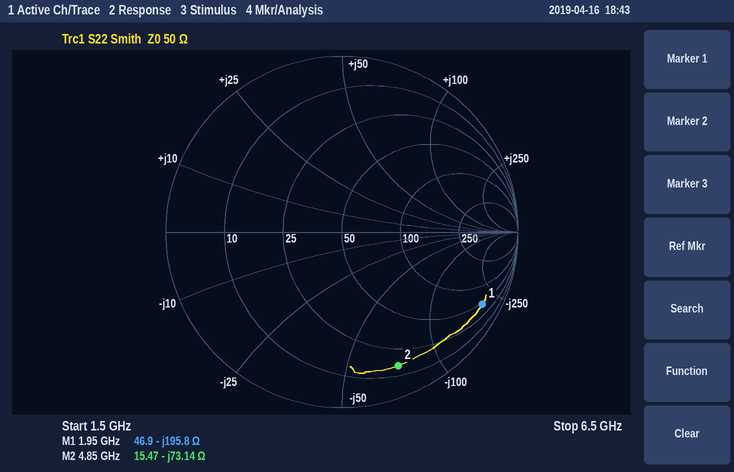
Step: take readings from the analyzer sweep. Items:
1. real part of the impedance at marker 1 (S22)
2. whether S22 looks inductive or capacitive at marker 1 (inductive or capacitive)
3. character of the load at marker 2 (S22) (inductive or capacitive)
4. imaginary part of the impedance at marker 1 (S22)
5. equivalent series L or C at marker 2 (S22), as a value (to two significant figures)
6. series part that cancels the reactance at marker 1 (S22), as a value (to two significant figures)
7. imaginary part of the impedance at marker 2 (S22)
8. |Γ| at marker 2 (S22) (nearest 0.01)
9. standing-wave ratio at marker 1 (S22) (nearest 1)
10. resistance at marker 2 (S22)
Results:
46.9 Ω
capacitive
capacitive
-195.8 Ω
450 fF
16 nH
-73.14 Ω
0.82
18
15.47 Ω
